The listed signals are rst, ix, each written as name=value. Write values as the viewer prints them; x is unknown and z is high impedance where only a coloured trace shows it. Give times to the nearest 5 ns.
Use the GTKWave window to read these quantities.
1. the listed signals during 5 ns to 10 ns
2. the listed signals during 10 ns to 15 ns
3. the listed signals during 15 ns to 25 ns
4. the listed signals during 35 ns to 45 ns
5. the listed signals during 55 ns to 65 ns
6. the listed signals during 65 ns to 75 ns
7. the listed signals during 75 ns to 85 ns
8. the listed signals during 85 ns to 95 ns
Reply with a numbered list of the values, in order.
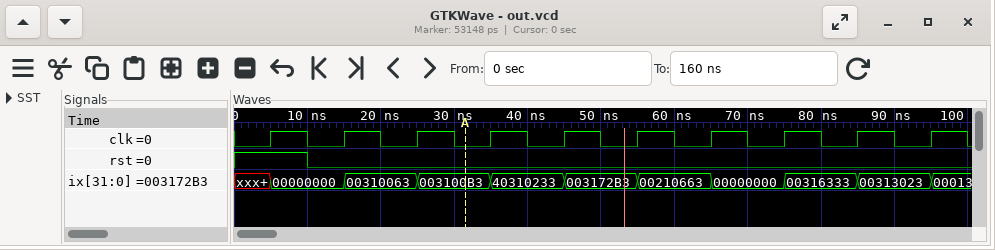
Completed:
1. rst=1, ix=00000000
2. rst=0, ix=00000000
3. rst=0, ix=00310063
4. rst=0, ix=40310233
5. rst=0, ix=00210663
6. rst=0, ix=00000000
7. rst=0, ix=00316333
8. rst=0, ix=00313023
